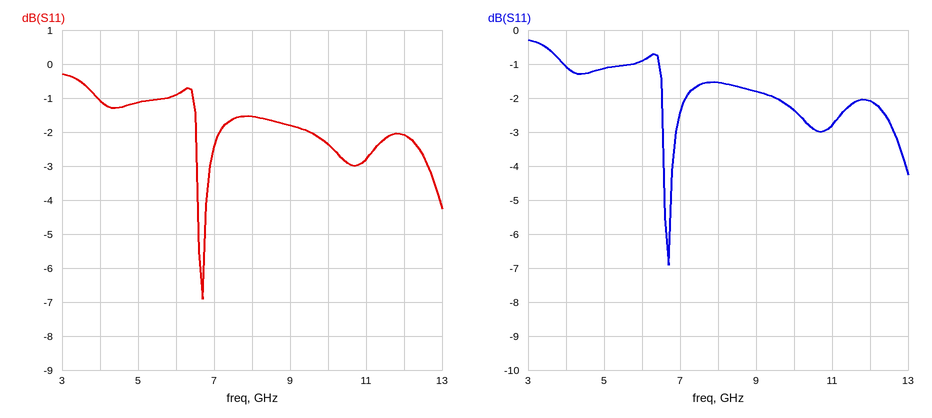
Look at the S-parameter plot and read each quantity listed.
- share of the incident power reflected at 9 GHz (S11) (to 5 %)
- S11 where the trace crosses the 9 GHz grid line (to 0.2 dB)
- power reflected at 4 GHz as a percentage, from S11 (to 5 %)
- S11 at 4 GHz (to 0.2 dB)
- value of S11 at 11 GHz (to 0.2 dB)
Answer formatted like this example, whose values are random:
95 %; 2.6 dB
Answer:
65 %; -1.8 dB; 80 %; -1.0 dB; -2.8 dB
